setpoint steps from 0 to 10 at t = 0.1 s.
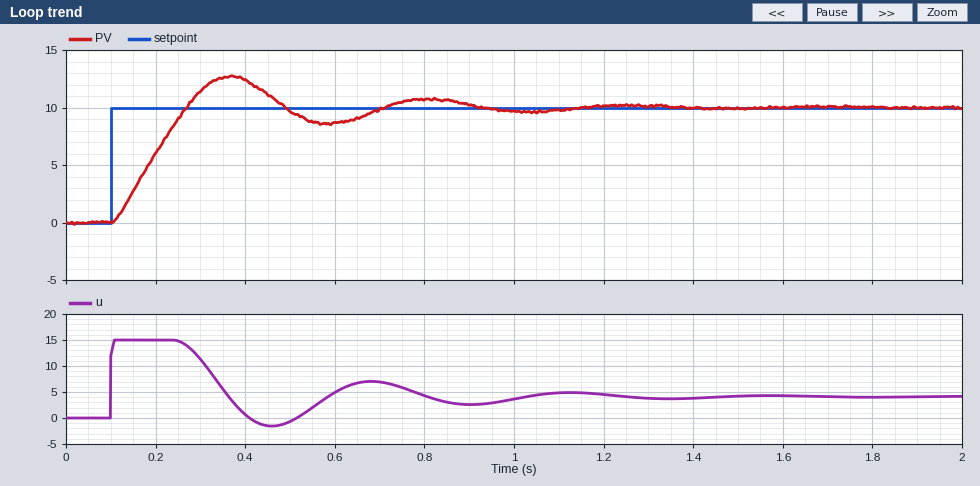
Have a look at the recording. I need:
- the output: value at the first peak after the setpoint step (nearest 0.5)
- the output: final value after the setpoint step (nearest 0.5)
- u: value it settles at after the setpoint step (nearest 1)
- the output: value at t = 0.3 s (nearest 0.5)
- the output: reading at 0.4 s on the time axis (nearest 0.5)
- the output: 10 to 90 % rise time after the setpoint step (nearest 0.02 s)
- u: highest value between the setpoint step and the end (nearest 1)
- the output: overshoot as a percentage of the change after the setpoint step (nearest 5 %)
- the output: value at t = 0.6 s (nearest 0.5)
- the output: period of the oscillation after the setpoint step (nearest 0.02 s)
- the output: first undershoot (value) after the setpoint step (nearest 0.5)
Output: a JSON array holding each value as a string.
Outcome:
["12.5", "10.0", "4", "11.5", "12.5", "0.12 s", "15", "25 %", "8.5", "0.44 s", "8.5"]
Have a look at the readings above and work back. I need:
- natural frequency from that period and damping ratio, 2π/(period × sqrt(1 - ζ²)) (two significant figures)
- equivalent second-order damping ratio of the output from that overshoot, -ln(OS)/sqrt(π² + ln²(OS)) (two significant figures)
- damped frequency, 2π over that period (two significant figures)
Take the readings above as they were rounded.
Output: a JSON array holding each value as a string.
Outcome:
["16 rad/s", "0.40", "14 rad/s"]
